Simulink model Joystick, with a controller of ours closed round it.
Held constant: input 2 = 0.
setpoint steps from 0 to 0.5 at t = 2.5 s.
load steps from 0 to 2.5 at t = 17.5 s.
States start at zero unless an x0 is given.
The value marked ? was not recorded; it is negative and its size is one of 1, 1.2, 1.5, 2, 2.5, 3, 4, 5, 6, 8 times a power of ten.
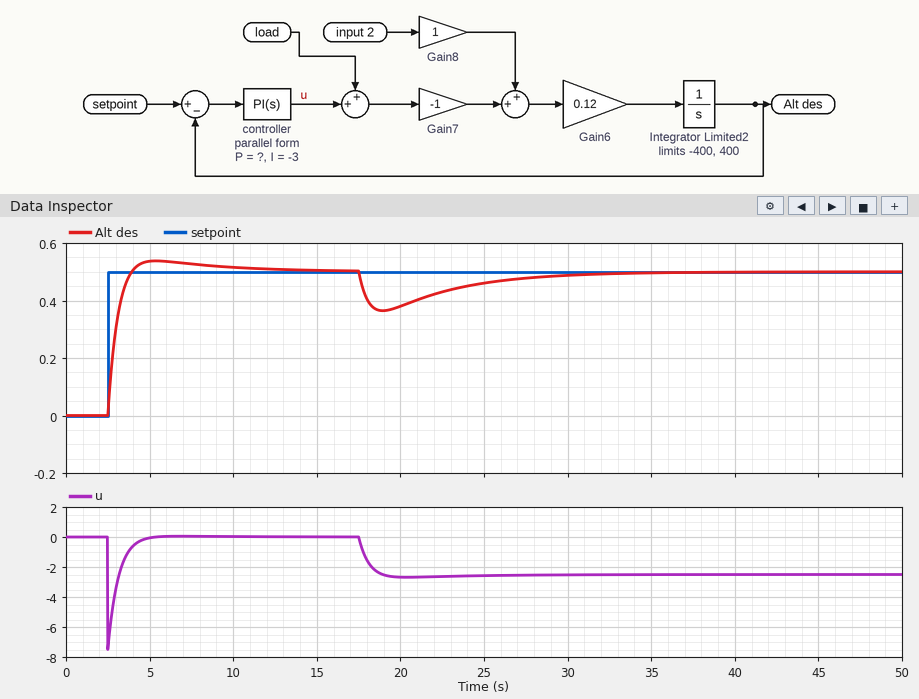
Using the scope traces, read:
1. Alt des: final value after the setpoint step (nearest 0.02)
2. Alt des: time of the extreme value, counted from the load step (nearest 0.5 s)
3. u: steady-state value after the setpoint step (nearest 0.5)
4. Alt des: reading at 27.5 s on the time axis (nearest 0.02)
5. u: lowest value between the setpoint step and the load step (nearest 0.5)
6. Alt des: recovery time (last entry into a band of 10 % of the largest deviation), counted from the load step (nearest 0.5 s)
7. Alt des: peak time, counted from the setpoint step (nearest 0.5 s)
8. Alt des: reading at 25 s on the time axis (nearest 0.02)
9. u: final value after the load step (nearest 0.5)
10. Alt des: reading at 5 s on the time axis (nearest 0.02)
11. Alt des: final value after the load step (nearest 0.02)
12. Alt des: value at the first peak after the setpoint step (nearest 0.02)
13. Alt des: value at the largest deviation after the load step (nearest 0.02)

0.50
1.5 s
0.0
0.48
-7.5
12.0 s
3.0 s
0.46
-2.5
0.54
0.50
0.54
0.36
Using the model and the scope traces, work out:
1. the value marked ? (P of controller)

-15
